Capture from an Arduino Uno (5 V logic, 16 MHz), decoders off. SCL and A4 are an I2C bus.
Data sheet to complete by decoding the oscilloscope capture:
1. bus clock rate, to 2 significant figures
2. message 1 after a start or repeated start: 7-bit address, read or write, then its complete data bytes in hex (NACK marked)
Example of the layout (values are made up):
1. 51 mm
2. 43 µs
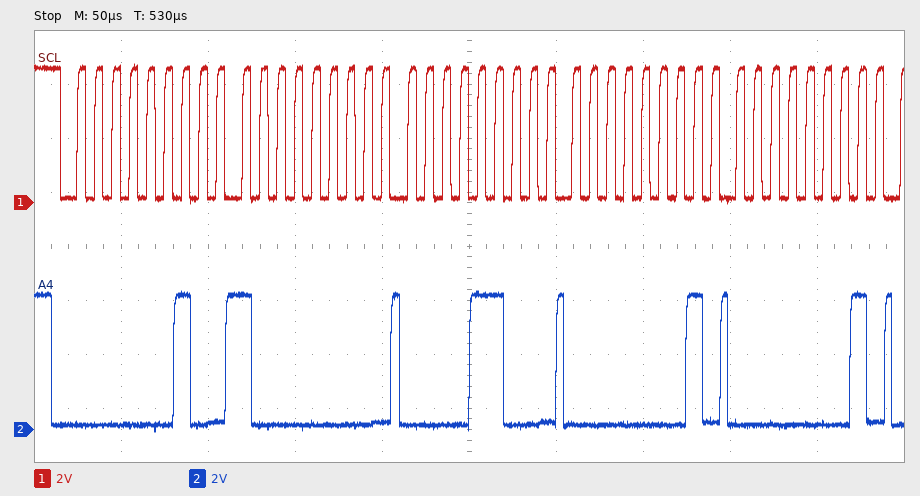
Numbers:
1. 100 kHz
2. 0x01 write: 80 0C 01 01
